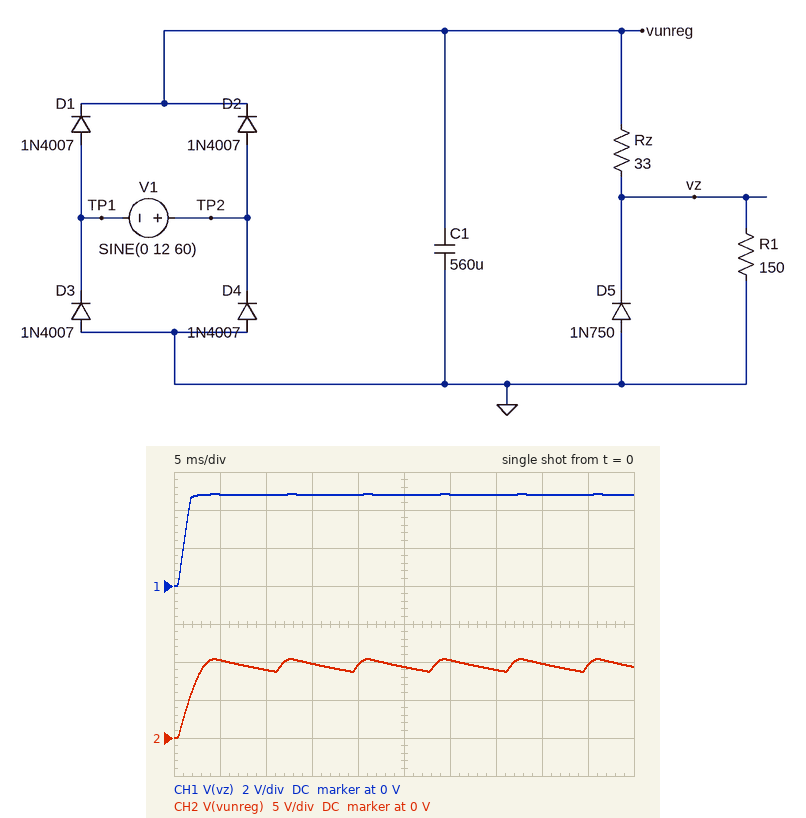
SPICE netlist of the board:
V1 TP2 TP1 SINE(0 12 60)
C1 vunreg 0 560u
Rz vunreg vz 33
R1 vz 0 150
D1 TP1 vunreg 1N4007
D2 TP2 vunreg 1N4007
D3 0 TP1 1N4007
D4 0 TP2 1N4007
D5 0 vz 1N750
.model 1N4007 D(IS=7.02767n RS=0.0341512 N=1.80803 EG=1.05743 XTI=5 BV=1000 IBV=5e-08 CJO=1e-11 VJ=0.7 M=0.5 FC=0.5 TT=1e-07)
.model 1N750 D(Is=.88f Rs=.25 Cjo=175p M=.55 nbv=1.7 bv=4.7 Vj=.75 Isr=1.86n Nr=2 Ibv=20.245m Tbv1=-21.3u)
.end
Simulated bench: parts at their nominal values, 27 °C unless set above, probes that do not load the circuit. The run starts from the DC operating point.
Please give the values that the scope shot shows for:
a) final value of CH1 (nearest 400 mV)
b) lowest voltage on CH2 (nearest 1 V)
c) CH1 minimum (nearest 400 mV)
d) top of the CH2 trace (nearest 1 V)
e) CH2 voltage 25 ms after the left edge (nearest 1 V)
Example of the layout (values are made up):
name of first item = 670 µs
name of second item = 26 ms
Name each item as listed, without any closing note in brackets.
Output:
final value of CH1 = 4.8 V
lowest voltage on CH2 = 0 V
CH1 minimum = 0 V
top of the CH2 trace = 10 V
CH2 voltage 25 ms after the left edge = 9 V
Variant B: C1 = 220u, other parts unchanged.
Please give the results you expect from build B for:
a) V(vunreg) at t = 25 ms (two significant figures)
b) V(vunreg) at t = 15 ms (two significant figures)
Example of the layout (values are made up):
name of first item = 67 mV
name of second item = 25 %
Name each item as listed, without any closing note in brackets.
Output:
V(vunreg) at t = 25 ms = 8.1 V
V(vunreg) at t = 15 ms = 9.0 V
